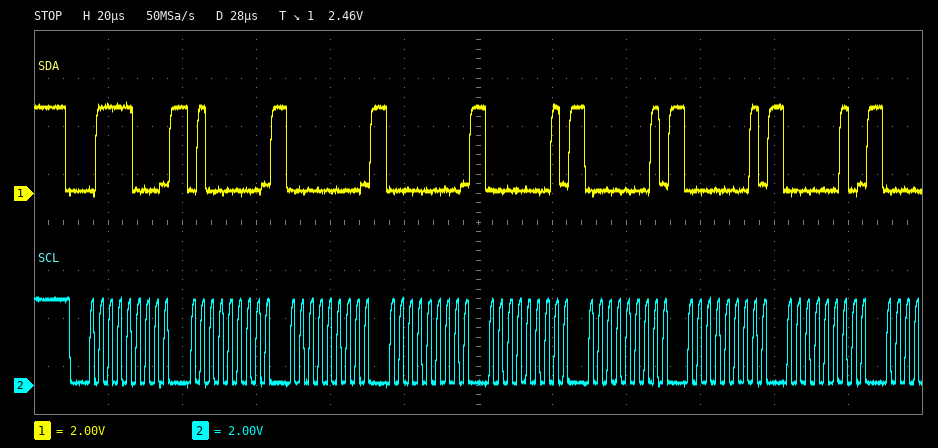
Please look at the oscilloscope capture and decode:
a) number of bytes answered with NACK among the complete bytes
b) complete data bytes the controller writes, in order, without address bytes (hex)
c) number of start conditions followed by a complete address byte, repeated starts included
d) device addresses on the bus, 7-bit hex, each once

0
40 00 00 01 01 01 02
1
0x3C
